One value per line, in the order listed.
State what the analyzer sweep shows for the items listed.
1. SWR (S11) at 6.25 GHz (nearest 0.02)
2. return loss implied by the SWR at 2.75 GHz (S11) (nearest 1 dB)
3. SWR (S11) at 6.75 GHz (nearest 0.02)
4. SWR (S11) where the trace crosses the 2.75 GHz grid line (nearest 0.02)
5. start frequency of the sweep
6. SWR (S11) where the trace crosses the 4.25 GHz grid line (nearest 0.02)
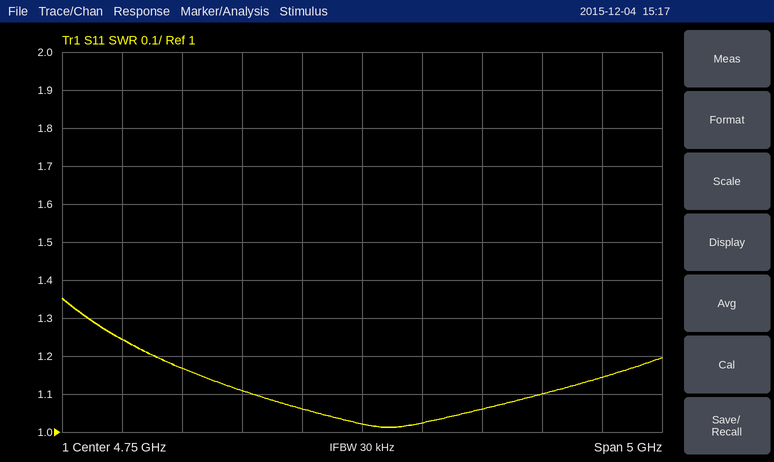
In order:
1.10
19 dB
1.14
1.24
2.25 GHz
1.06
